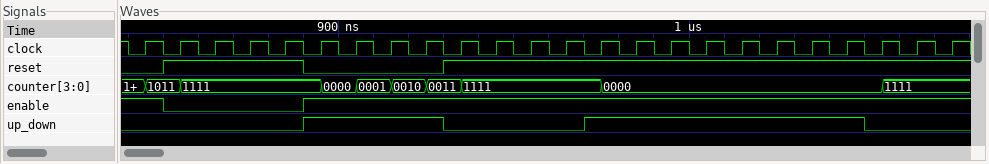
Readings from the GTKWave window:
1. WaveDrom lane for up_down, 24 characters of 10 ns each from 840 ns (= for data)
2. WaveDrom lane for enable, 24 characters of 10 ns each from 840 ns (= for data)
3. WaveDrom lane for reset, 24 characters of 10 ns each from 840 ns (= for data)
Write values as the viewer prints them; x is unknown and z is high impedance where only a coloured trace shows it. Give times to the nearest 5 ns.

{name: 'up_down', wave: '0....1...0...1.......0..'}
{name: 'enable', wave: '10...1..................'}
{name: 'reset', wave: '01...0...1..............'}
